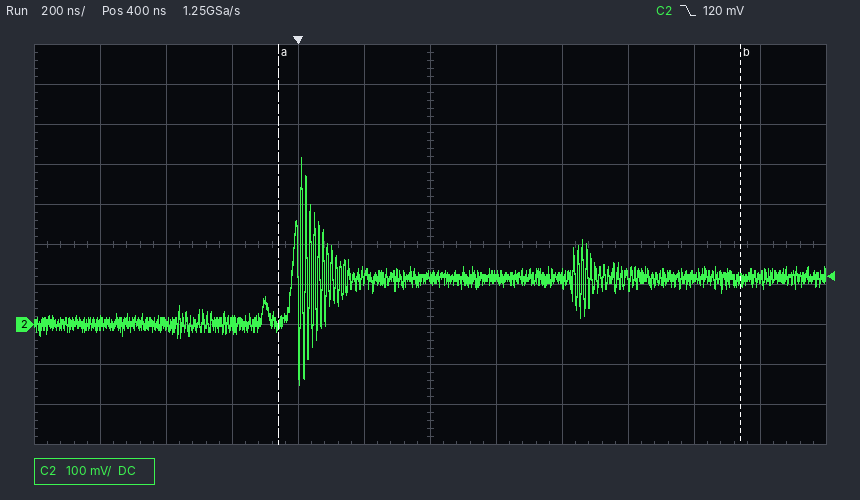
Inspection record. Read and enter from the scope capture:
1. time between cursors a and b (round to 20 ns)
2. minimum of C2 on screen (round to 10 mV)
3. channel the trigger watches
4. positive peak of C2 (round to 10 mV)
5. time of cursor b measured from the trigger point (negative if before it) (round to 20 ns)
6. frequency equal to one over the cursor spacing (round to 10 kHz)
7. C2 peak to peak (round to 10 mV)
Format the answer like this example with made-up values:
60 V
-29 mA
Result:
1.40 µs
-150 mV
C2
420 mV
+1.34 µs
710 kHz
570 mV
